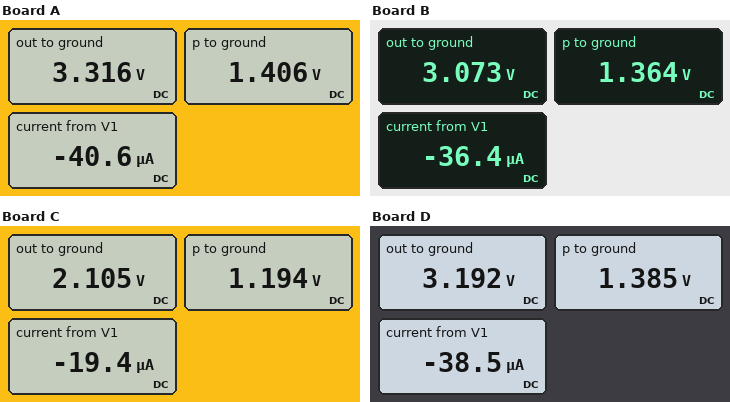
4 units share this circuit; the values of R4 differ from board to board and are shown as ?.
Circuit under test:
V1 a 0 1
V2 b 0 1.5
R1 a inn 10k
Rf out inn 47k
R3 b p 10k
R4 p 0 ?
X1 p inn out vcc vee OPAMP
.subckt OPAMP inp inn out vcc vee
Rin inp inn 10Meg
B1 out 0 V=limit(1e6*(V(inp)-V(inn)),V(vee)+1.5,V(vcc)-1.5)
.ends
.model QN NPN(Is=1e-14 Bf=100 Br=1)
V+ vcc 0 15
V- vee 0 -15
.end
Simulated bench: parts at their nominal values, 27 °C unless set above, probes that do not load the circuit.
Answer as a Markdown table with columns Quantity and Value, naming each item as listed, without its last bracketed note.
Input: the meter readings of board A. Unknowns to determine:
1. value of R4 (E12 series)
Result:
| Quantity | Value |
|---|---|
| value of R4 | 150 kΩ |
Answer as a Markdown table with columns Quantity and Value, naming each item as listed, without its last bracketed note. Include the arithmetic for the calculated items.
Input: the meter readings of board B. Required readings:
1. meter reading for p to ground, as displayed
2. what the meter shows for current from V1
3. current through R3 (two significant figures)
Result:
| Quantity | Value |
|---|---|
| meter reading for p to ground, as displayed | 1.364 V |
| what the meter shows for current from V1 | -36.4 µA |
| current through R3 | (1.5 V - 1.364 V) / 10 kΩ = 14 µA |
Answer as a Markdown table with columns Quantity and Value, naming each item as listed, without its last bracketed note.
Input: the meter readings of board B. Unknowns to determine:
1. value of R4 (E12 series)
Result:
| Quantity | Value |
|---|---|
| value of R4 | 100 kΩ |
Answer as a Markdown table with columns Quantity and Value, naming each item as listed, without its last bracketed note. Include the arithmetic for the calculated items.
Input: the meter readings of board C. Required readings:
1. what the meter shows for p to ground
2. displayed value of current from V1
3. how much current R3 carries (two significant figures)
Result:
| Quantity | Value |
|---|---|
| what the meter shows for p to ground | 1.194 V |
| displayed value of current from V1 | -19.4 µA |
| how much current R3 carries | (1.5 V - 1.194 V) / 10 kΩ = 31 µA |
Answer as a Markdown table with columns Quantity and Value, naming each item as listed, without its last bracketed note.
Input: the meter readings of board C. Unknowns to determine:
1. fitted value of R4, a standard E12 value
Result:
| Quantity | Value |
|---|---|
| fitted value of R4, a standard E12 value | 39 kΩ |
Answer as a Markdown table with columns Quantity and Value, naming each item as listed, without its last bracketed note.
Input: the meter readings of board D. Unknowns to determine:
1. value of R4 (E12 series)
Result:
| Quantity | Value |
|---|---|
| value of R4 | 120 kΩ |
